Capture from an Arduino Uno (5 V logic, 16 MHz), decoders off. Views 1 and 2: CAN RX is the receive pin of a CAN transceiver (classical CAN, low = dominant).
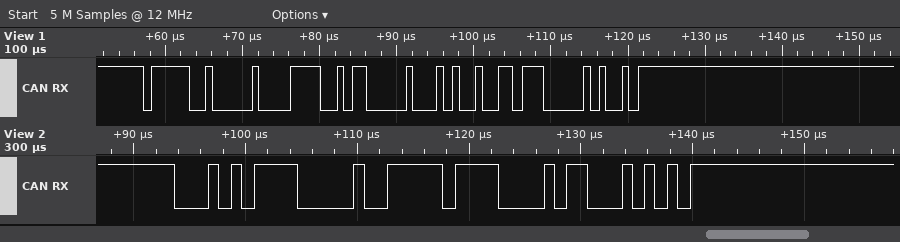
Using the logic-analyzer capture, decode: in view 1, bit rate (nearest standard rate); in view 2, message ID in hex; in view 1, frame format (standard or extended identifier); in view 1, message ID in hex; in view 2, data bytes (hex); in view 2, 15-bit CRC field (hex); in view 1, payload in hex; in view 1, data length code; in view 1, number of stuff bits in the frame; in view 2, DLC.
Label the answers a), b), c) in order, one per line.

a) 1000 kbit/s
b) 0x15E
c) standard
d) 0x7D0
e) FF
f) 0x058A
g) CB 00 A4
h) 3
i) 4
j) 1
